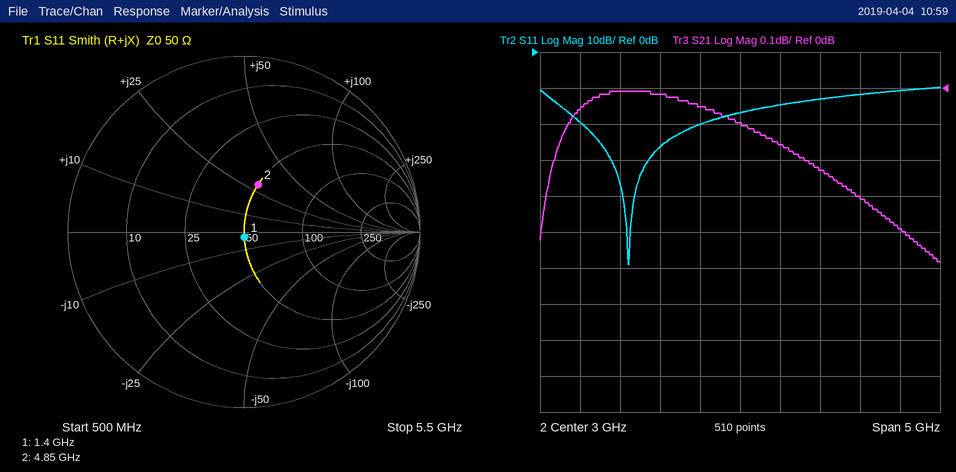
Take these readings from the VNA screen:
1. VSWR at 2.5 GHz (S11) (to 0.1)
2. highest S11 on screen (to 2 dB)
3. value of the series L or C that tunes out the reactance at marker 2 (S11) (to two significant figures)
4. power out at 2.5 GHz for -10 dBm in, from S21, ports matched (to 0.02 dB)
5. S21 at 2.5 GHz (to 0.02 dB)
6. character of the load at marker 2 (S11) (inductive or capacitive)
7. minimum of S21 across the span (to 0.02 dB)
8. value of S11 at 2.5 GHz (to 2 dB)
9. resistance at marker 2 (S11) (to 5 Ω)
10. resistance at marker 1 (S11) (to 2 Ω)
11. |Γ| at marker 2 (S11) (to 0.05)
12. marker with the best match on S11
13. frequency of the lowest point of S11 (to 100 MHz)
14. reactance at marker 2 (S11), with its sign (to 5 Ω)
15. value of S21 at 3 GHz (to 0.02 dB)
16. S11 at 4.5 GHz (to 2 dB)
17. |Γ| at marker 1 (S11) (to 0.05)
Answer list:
1.2
-10 dB
1.1 pF
-10.06 dBm
-0.06 dB
inductive
-0.48 dB
-20 dB
50 Ω
50 Ω
0.30
marker 1
1.6 GHz
+30 Ω
-0.10 dB
-12 dB
0.05
